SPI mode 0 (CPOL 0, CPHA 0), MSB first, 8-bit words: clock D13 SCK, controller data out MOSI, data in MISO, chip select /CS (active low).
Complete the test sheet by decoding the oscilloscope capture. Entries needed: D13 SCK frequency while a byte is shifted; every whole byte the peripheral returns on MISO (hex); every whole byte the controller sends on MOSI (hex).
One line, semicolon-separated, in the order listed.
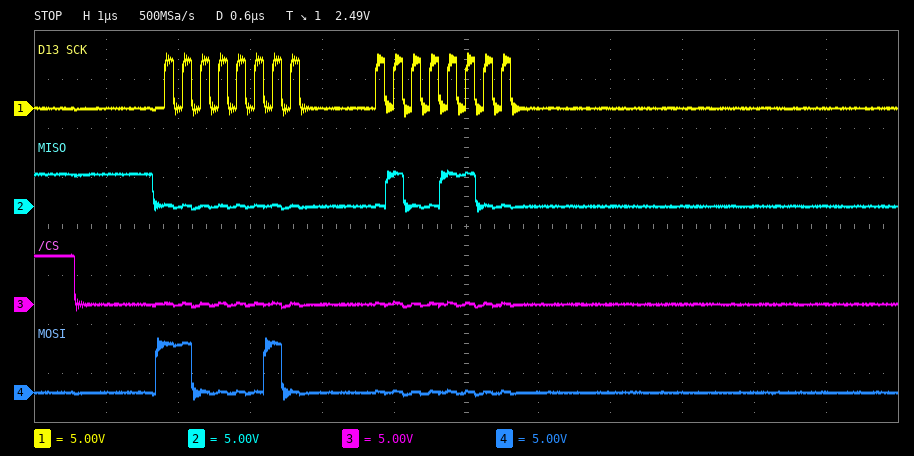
4 MHz; 0x00 0x4C; 0xC2 0x00
